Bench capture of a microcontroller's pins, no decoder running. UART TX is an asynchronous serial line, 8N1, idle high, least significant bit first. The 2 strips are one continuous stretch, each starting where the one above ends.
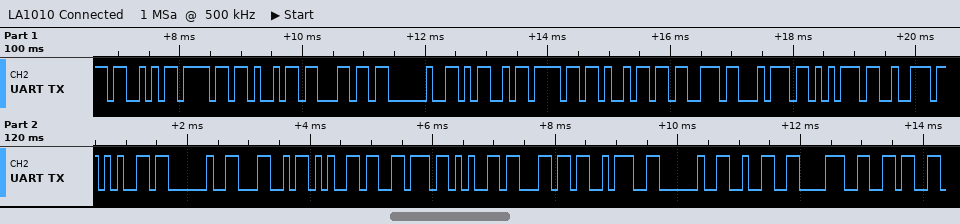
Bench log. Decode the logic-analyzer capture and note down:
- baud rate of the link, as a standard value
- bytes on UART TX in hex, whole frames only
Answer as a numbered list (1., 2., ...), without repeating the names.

1. 9600 baud
2. 53 6F 69 6C 20 4D 6F 69 73 74 75 72 65 20 4C 65 76 65 6C 3A 20 32 38 36
